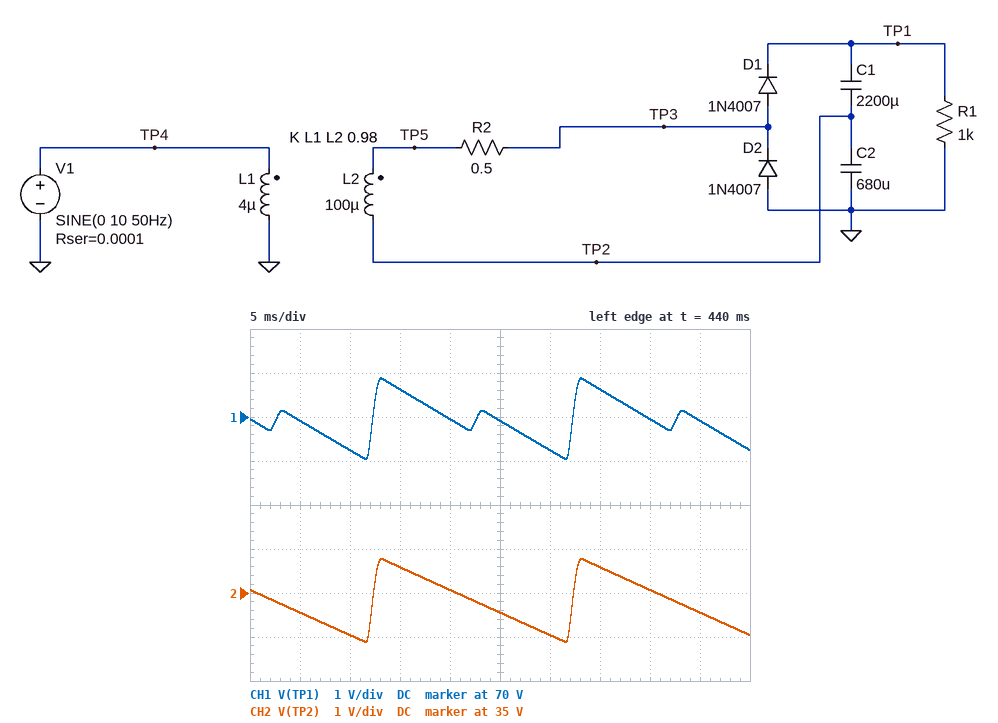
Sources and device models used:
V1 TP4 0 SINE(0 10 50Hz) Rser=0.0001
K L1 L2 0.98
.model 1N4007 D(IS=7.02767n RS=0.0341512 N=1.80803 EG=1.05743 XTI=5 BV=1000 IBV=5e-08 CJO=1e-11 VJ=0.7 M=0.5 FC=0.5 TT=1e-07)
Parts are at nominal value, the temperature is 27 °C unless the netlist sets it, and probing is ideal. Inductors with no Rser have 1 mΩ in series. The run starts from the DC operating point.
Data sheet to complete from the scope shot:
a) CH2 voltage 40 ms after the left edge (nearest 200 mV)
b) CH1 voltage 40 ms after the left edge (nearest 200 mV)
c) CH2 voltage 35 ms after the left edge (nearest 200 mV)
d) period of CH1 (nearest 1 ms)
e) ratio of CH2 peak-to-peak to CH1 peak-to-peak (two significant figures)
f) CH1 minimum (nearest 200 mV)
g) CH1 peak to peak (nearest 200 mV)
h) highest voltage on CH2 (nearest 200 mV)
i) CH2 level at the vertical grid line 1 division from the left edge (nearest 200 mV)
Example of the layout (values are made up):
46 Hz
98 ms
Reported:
35.0 V
70.0 V
35.6 V
20 ms
1.0
69.0 V
1.8 V
35.8 V
34.6 V
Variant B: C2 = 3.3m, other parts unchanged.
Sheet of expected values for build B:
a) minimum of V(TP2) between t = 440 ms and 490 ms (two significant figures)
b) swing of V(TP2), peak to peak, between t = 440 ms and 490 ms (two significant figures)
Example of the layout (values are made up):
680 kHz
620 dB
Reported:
35 V
390 mV
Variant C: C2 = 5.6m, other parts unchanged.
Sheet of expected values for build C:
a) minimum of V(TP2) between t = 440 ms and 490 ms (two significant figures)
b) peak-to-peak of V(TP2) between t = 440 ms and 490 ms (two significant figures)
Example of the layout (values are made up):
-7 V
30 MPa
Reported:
35 V
230 mV
